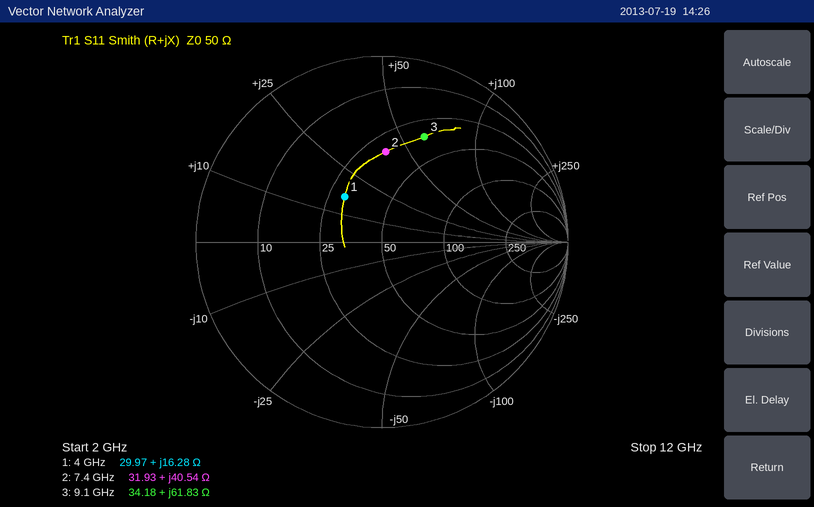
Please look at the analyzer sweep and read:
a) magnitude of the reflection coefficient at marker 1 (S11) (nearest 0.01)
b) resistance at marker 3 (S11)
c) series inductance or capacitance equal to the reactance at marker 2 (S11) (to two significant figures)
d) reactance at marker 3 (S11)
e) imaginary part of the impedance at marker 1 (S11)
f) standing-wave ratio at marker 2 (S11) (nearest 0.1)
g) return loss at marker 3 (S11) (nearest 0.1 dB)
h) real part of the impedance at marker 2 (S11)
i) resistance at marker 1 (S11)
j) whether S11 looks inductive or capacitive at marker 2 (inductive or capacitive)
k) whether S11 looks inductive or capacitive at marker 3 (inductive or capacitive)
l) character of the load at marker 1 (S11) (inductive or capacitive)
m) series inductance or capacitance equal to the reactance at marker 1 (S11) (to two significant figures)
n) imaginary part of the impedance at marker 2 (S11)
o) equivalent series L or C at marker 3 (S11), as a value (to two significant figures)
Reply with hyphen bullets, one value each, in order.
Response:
- 0.32
- 34.18 Ω
- 870 pH
- +61.83 Ω
- +16.28 Ω
- 2.9
- 4.3 dB
- 31.93 Ω
- 29.97 Ω
- inductive
- inductive
- inductive
- 650 pH
- +40.54 Ω
- 1.1 nH
